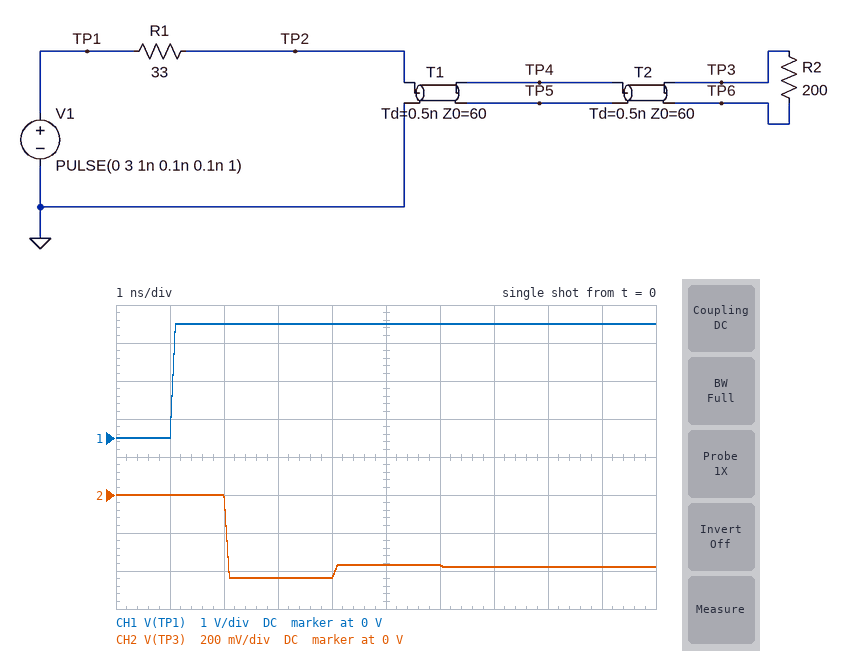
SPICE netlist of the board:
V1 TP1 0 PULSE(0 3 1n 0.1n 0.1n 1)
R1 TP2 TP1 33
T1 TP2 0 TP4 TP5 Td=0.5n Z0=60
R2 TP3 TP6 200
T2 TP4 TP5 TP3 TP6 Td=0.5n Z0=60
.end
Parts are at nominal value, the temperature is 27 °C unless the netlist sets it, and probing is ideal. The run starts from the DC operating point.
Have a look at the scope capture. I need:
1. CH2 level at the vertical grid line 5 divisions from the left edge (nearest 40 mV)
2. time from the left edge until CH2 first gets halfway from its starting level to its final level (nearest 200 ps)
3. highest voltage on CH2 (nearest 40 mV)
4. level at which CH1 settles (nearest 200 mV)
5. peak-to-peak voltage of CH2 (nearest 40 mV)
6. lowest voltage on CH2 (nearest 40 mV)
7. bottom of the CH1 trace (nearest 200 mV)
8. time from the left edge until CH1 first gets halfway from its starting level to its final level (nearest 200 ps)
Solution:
-360 mV
2.0 ns
0 V
3.0 V
440 mV
-440 mV
0 V
1.0 ns
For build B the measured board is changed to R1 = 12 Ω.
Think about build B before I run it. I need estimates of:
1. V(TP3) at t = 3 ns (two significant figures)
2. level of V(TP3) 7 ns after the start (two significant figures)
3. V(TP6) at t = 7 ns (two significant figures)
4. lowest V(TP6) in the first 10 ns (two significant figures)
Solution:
-570 mV
-440 mV
-3.4 V
-4.4 V
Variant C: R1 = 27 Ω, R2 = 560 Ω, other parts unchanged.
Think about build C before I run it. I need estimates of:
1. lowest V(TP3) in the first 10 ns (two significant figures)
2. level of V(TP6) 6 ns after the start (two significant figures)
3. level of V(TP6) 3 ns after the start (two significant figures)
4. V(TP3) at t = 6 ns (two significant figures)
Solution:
-200 mV
-2.7 V
-3.9 V
-140 mV
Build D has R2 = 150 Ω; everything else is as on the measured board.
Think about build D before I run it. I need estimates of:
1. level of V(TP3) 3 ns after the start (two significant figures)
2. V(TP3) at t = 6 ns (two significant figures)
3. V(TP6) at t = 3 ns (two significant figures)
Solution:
-540 mV
-480 mV
-3.3 V
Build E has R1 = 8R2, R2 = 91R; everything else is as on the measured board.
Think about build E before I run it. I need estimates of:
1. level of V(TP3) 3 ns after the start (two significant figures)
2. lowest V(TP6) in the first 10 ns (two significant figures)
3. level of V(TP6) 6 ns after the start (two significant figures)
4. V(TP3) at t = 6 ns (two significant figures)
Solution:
-1.0 V
-4.2 V
-3.6 V
-870 mV
